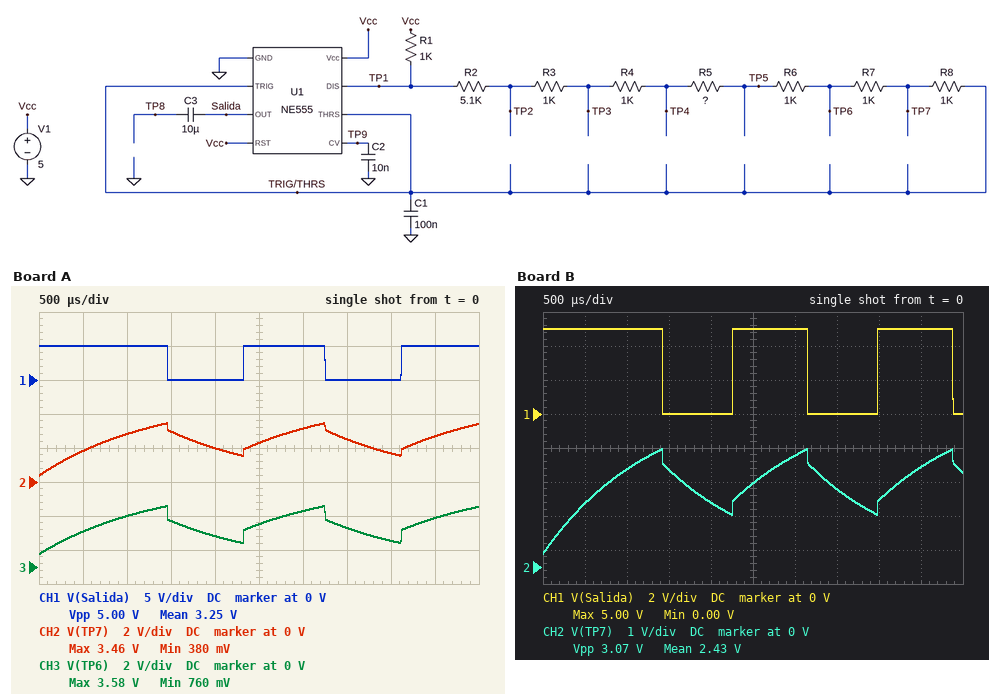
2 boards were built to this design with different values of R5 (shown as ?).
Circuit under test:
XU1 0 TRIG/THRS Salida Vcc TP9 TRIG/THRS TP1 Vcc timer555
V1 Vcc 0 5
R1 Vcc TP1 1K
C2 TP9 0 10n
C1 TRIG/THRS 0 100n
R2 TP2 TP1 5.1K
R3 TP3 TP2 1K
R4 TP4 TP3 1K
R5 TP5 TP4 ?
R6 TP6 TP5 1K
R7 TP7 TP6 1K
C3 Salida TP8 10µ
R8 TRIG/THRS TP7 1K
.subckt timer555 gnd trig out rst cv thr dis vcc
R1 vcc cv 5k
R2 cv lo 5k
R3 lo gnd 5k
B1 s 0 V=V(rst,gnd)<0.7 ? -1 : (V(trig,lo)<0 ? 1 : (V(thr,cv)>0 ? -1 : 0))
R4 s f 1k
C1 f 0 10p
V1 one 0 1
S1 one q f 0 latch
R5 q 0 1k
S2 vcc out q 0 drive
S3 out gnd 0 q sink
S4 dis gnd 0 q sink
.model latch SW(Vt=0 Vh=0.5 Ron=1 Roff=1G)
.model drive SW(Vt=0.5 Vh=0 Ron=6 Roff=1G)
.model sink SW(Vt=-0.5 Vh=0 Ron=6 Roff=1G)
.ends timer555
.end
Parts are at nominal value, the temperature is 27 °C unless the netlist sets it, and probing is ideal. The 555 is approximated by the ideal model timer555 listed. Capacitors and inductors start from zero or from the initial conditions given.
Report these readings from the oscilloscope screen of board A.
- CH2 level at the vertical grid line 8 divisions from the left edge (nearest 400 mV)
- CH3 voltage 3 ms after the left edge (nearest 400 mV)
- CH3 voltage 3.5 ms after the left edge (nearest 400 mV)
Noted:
1.6 V
3.2 V
2.4 V
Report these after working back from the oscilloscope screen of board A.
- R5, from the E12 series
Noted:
2.2 kΩ
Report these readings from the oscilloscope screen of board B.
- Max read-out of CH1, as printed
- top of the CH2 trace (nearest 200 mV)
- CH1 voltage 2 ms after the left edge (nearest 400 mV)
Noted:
5.00 V
3.4 V
0 V
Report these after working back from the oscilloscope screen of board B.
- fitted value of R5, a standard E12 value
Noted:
1.8 kΩ
